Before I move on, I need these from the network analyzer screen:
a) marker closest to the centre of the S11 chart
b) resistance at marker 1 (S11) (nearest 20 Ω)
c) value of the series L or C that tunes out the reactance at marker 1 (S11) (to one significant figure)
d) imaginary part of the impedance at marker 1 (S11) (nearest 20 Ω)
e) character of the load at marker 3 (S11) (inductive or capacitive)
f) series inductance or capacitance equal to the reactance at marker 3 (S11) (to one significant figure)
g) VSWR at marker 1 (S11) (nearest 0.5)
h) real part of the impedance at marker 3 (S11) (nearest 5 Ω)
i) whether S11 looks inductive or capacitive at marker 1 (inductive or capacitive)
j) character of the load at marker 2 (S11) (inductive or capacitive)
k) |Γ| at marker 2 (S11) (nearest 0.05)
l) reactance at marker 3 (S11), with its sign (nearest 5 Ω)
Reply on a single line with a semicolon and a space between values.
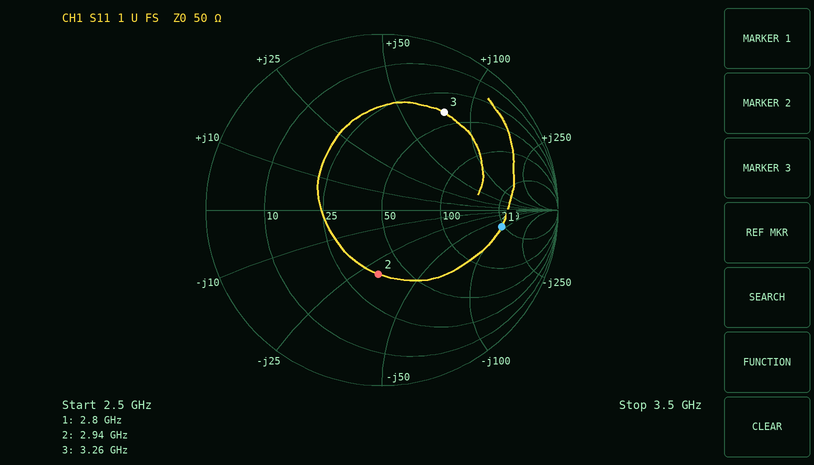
marker 2; 240 Ω; 5 nH; -80 Ω; inductive; 4 nH; 5.5; 40 Ω; capacitive; capacitive; 0.35; +75 Ω
